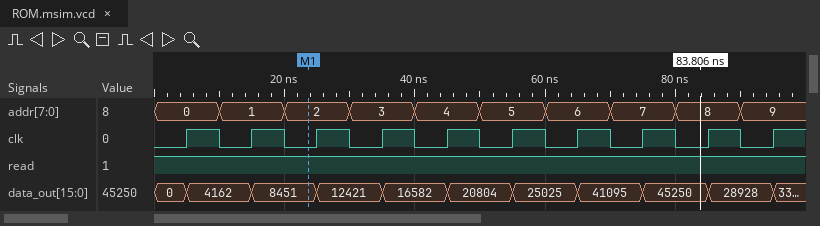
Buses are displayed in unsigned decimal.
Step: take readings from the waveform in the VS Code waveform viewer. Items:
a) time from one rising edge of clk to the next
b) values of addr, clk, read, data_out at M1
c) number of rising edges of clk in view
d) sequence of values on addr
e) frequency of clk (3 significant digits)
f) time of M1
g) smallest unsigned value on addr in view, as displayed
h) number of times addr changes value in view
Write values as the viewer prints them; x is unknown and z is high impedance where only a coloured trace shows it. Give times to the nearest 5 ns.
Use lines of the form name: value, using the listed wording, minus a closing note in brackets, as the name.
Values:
time from one rising edge of clk to the next: 10 ns
values of addr, clk, read, data_out at M1: addr=2, clk=0, read=1, data_out=8451
number of rising edges of clk in view: 10
sequence of values on addr: 0, 1, 2, 3, 4, 5, 6, 7, 8, 9
frequency of clk: 100 MHz
time of M1: 25 ns
smallest unsigned value on addr in view, as displayed: 0
number of times addr changes value in view: 9
